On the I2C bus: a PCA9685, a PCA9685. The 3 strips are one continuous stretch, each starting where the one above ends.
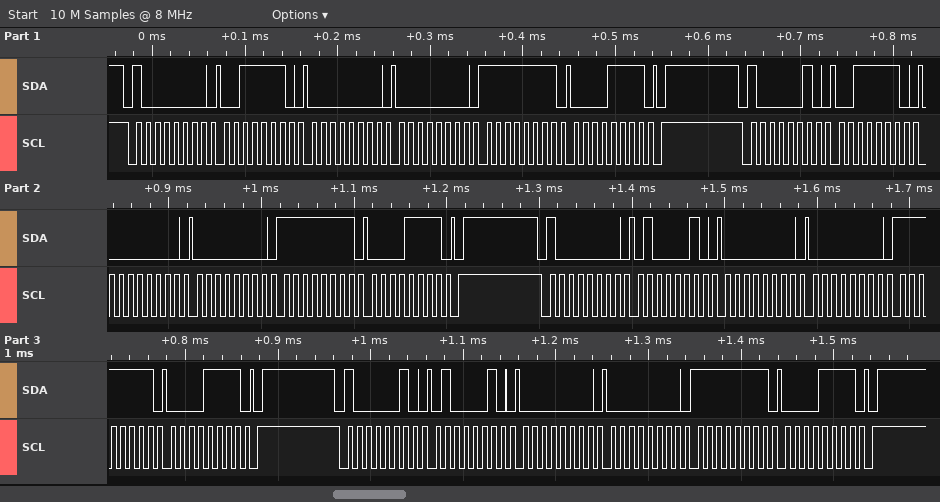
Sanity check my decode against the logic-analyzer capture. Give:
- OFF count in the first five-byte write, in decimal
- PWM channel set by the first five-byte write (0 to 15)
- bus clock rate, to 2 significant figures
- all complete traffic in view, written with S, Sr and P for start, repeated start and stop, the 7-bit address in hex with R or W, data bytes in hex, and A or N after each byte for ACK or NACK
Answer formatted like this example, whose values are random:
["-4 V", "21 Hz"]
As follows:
["4095", "14", "100 kHz", "S 40W A 3E A 00 A 00 A FF A 0F A P S 41W A 3E A 00 A 00 A FF A 0F A P S 40W A 42 A 00 A 00 A FF A 0F A P S 41W A 42 A 00 A 00 A FF A 0F A P"]
